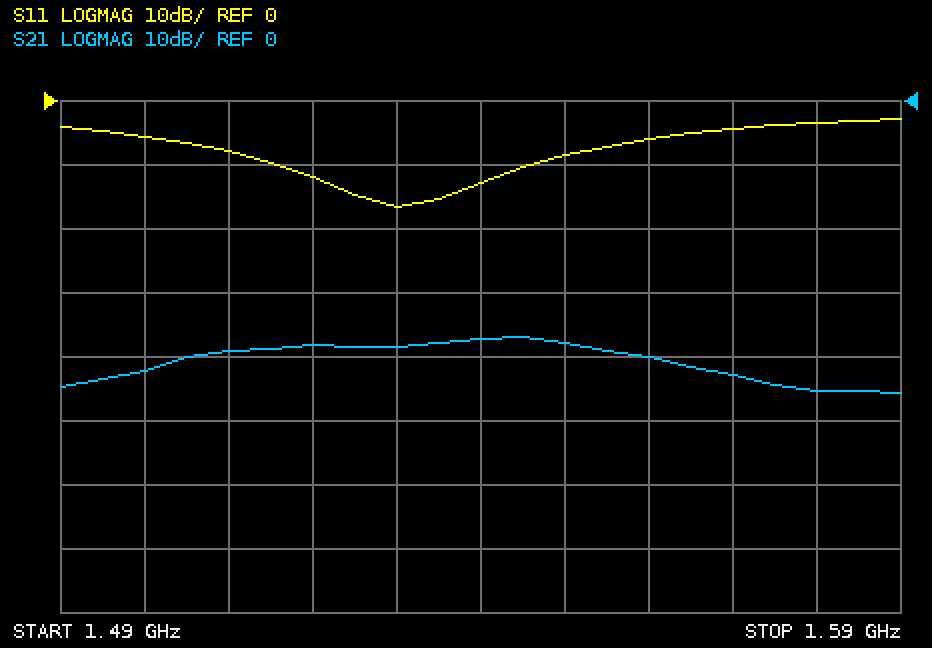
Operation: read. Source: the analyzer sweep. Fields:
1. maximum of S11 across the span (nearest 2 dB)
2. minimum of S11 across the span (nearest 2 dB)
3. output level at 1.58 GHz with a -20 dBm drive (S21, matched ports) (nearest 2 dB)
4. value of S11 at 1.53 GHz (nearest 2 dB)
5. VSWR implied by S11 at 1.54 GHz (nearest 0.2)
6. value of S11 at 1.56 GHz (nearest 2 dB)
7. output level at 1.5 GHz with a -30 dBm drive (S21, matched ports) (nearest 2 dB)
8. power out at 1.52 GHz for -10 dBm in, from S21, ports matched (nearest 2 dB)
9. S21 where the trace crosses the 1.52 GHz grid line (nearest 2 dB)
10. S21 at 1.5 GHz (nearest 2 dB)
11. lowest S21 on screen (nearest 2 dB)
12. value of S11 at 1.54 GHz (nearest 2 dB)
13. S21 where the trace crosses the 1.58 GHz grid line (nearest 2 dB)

-2 dB
-16 dB
-66 dBm
-16 dB
1.6
-6 dB
-72 dBm
-48 dBm
-38 dB
-42 dB
-46 dB
-12 dB
-46 dB
